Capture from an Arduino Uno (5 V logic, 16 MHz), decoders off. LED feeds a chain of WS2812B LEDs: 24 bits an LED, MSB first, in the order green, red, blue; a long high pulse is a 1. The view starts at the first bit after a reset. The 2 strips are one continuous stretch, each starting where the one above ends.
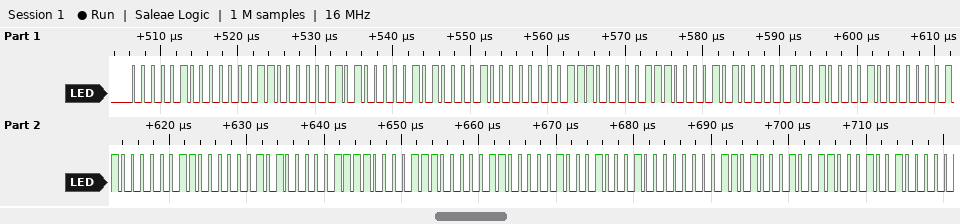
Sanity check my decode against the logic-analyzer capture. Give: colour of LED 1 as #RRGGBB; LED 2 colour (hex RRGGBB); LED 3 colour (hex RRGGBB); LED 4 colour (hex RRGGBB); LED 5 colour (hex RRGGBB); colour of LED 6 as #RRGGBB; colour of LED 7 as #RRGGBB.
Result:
#060405
#080507
#0A0709
#0C080C
#0F0A0E
#110C10
#130D12
